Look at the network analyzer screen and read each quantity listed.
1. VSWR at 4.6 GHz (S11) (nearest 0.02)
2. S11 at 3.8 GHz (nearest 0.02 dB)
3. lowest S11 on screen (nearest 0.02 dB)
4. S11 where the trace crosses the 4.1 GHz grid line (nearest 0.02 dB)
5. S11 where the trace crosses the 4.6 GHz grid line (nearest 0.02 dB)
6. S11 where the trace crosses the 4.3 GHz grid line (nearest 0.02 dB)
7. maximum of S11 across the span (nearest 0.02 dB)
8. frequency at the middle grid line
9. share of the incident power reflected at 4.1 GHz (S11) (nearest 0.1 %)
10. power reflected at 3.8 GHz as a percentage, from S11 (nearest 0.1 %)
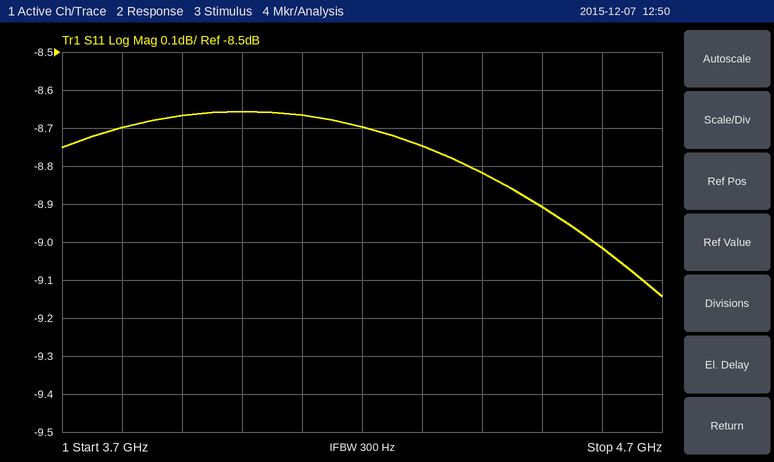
2.10
-8.70 dB
-9.14 dB
-8.66 dB
-9.02 dB
-8.74 dB
-8.66 dB
4.2 GHz
13.6 %
13.5 %
